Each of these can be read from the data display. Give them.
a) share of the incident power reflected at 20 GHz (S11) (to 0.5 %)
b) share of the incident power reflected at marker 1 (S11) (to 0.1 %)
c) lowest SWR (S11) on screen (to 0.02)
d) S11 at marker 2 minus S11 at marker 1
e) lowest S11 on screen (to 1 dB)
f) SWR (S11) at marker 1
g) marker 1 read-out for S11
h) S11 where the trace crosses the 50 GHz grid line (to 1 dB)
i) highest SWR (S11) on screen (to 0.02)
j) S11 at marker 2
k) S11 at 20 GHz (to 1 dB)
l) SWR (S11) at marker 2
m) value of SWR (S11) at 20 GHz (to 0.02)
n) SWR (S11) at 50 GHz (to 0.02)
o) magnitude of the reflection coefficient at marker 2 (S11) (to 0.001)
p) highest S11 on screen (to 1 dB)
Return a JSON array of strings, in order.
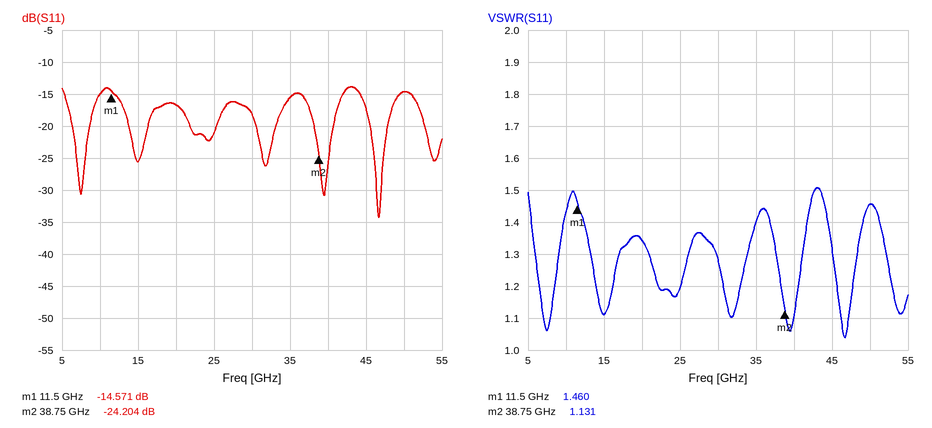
["2.0 %", "3.5 %", "1.04", "-9.633 dB", "-34 dB", "1.460", "-14.571 dB", "-15 dB", "1.50", "-24.204 dB", "-17 dB", "1.131", "1.34", "1.46", "0.062", "-14 dB"]
